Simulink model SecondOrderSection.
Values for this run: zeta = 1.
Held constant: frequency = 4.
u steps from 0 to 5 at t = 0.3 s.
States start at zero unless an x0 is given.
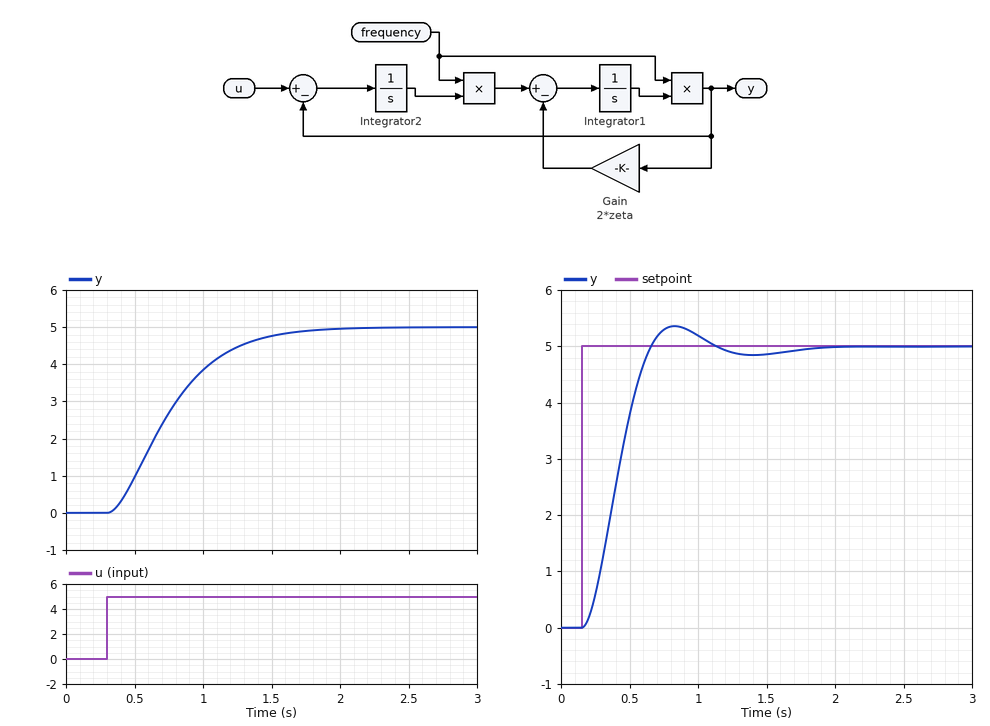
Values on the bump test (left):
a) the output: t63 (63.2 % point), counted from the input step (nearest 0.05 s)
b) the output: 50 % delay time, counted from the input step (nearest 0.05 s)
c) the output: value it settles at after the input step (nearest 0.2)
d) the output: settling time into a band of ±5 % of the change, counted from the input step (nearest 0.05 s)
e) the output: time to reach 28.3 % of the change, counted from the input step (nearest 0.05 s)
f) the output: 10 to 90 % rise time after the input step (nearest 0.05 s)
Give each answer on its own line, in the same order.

0.55 s
0.40 s
5.0
1.20 s
0.25 s
0.85 s
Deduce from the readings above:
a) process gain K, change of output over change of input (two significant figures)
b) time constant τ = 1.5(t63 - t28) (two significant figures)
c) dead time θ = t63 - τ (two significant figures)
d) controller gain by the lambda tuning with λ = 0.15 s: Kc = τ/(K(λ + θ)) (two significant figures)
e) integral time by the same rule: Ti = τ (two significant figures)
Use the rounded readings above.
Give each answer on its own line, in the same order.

1.0
0.45 s
0.10 s
1.8
0.45 s
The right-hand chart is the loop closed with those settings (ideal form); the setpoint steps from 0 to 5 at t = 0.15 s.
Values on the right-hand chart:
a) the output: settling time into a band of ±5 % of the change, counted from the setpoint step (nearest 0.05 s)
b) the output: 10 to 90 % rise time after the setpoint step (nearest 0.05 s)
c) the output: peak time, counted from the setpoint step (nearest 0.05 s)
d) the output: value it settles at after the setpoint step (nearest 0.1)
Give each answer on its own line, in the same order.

0.80 s
0.35 s
0.70 s
5.0
